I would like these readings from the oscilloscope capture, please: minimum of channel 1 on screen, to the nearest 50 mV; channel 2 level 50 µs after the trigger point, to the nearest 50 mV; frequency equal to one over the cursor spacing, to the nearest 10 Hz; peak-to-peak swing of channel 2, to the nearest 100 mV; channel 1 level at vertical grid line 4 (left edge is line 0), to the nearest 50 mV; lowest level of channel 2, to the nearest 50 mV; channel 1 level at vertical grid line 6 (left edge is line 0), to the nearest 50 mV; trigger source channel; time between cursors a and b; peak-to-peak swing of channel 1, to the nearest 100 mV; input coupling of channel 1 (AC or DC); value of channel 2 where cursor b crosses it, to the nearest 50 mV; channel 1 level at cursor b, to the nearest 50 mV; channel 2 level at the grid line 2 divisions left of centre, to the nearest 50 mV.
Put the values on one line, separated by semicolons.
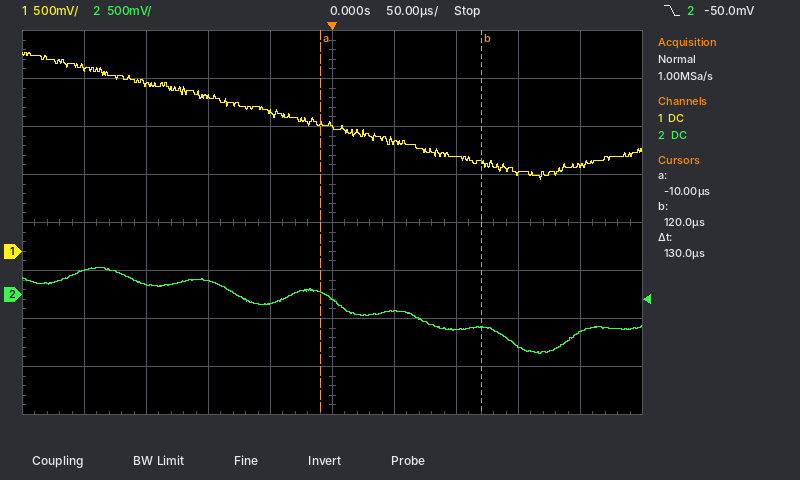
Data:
750 mV; -150 mV; 7.69 kHz; 900 mV; 1.45 V; -600 mV; 1.15 V; channel 2; 130 µs; 1.30 V; DC; -350 mV; 900 mV; 150 mV
